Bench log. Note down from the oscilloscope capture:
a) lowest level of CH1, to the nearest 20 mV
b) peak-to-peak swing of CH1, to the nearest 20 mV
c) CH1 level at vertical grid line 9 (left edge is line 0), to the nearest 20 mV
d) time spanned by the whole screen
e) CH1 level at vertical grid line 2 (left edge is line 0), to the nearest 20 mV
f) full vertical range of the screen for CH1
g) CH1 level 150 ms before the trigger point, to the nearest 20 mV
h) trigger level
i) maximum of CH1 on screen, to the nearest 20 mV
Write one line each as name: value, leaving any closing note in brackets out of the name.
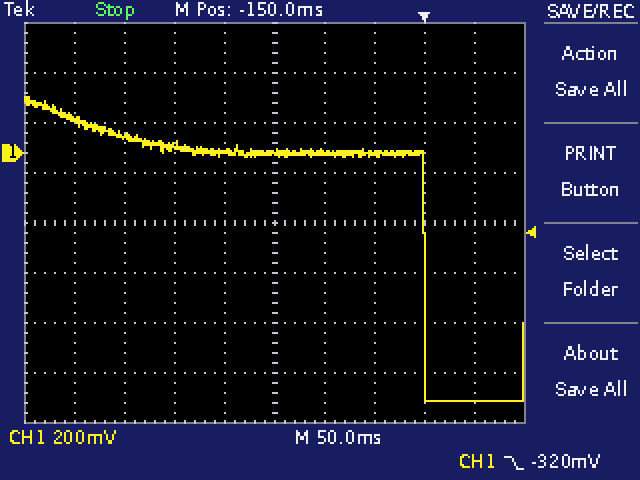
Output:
lowest level of CH1, to the nearest 20 mV: -1.00 V
peak-to-peak swing of CH1, to the nearest 20 mV: 1.22 V
CH1 level at vertical grid line 9 (left edge is line 0), to the nearest 20 mV: -1.00 V
time spanned by the whole screen: 500 ms
CH1 level at vertical grid line 2 (left edge is line 0), to the nearest 20 mV: 60 mV
full vertical range of the screen for CH1: 1.6 V
CH1 level 150 ms before the trigger point, to the nearest 20 mV: 0 mV
trigger level: -320 mV
maximum of CH1 on screen, to the nearest 20 mV: 220 mV
